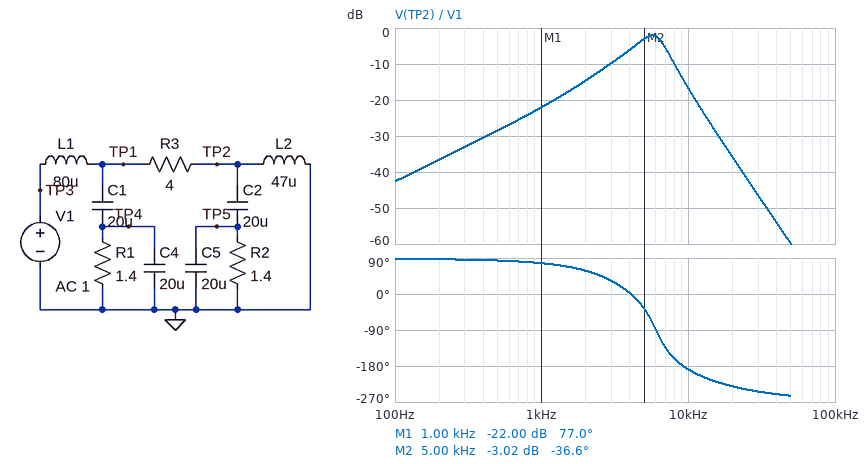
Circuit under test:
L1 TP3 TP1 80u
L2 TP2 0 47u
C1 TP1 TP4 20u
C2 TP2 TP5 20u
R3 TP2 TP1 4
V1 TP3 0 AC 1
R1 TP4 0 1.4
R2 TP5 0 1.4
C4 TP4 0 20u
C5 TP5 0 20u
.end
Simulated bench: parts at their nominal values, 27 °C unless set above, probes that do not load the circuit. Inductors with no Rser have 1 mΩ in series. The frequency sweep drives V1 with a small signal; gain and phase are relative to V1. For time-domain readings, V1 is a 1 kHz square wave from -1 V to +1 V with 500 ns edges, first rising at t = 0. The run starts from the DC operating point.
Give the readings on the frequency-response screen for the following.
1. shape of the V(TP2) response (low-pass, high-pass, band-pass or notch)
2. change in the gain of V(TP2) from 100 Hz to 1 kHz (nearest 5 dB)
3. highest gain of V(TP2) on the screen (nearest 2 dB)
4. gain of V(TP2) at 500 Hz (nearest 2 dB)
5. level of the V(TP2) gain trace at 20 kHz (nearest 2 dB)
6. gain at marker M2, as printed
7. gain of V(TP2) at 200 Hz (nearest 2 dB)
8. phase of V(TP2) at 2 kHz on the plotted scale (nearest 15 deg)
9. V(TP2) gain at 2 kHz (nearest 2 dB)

band-pass
20 dB
-2 dB
-28 dB
-36 dB
-3.02 dB
-36 dB
60 deg
-14 dB
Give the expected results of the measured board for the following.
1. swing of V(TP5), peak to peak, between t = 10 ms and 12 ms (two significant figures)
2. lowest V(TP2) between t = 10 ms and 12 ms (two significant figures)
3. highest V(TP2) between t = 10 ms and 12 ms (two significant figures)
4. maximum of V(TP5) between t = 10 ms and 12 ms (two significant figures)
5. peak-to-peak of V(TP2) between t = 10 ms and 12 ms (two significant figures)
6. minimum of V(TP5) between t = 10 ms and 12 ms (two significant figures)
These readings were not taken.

350 mV
-520 mV
520 mV
170 mV
1.0 V
-170 mV
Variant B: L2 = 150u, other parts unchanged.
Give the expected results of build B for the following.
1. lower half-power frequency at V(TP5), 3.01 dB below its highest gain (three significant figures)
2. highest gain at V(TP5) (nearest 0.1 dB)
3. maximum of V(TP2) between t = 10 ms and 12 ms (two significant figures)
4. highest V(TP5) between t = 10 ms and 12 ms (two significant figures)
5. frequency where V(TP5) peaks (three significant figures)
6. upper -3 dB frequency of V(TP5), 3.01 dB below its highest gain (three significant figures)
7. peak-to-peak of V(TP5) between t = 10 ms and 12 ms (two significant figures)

3.09 kHz
-5.1 dB
1.0 V
280 mV
4.06 kHz
5.01 kHz
550 mV
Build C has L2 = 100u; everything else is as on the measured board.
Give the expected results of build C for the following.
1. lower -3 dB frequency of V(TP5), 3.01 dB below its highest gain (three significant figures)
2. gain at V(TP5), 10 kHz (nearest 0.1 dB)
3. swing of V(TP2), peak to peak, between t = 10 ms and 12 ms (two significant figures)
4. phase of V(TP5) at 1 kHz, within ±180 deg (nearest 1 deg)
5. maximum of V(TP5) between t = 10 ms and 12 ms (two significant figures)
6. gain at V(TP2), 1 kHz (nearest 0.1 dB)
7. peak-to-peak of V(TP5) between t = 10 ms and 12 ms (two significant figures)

3.58 kHz
-25.2 dB
1.7 V
142 deg
260 mV
-15.3 dB
520 mV
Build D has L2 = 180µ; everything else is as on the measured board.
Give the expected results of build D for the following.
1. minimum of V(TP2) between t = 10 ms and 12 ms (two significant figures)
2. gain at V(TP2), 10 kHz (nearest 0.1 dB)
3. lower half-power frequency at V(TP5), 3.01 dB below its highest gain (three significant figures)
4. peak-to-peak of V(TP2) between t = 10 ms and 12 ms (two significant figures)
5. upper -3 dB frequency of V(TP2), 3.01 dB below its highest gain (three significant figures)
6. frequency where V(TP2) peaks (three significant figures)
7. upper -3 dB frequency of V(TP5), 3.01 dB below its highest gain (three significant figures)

-1.1 V
-19.6 dB
2.88 kHz
2.2 V
4.79 kHz
3.80 kHz
4.91 kHz
